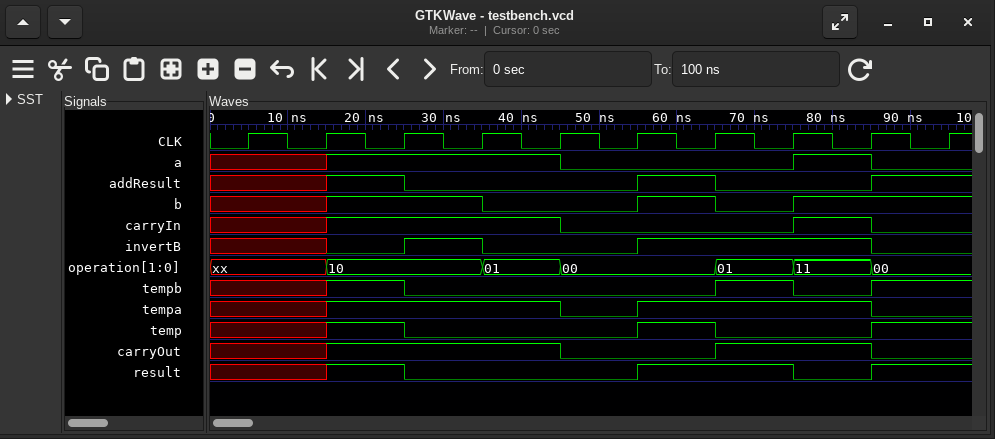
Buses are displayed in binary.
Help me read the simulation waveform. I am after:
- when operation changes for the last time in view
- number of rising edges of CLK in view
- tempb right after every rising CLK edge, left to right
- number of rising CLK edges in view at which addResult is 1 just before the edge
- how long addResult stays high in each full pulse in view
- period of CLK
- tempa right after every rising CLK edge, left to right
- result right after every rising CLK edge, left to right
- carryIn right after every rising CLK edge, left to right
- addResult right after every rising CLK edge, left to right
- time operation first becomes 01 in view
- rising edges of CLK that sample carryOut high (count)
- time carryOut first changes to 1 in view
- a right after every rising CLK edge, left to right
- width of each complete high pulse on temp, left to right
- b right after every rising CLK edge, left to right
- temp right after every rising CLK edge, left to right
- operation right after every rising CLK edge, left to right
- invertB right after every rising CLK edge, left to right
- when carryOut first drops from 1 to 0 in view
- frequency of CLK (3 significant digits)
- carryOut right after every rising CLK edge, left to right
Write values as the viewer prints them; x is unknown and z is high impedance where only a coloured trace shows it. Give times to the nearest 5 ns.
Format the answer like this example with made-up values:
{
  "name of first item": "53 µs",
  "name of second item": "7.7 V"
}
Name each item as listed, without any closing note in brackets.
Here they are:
{
  "when operation changes for the last time in view": "85 ns",
  "number of rising edges of CLK in view": "10",
  "tempb right after every rising CLK edge, left to right": "x 1 0 0 0 0 1 0 1 1",
  "number of rising CLK edges in view at which addResult is 1 just before the edge": "3",
  "how long addResult stays high in each full pulse in view": "10 ns",
  "period of CLK": "10 ns",
  "tempa right after every rising CLK edge, left to right": "x 1 1 1 0 1 1 1 0 0",
  "result right after every rising CLK edge, left to right": "x 1 0 0 0 1 1 0 1 1",
  "carryIn right after every rising CLK edge, left to right": "x 1 1 1 0 0 0 1 0 0",
  "addResult right after every rising CLK edge, left to right": "x 1 0 0 0 1 0 0 1 1",
  "time operation first becomes 01 in view": "35 ns",
  "rising edges of CLK that sample carryOut high": "5",
  "time carryOut first changes to 1 in view": "15 ns",
  "a right after every rising CLK edge, left to right": "x 1 1 1 0 0 0 1 0 0",
  "width of each complete high pulse on temp, left to right": "10 ns",
  "b right after every rising CLK edge, left to right": "x 1 1 0 0 1 0 1 1 1",
  "temp right after every rising CLK edge, left to right": "x 1 0 0 0 1 0 0 1 1",
  "operation right after every rising CLK edge, left to right": "xx, 10, 10, 01, 00, 00, 01, 11, 00, 00",
  "invertB right after every rising CLK edge, left to right": "x 0 1 0 0 1 1 1 0 0",
  "when carryOut first drops from 1 to 0 in view": "45 ns",
  "frequency of CLK": "100 MHz",
  "carryOut right after every rising CLK edge, left to right": "x 1 1 1 0 0 1 1 0 0"
}
